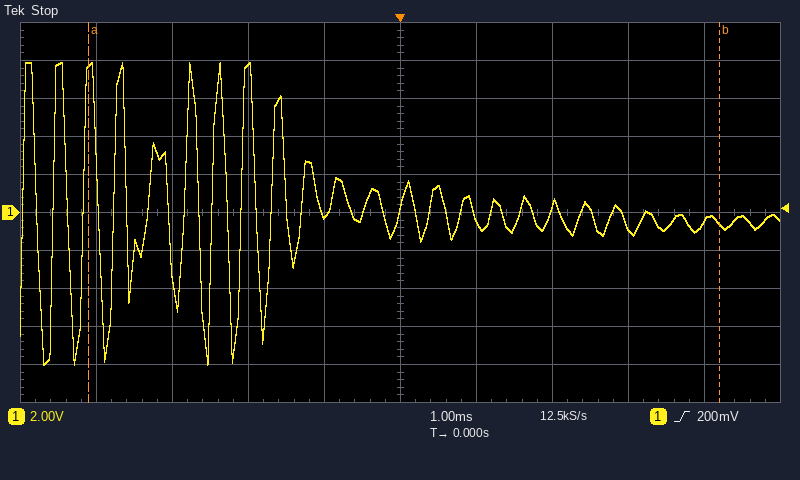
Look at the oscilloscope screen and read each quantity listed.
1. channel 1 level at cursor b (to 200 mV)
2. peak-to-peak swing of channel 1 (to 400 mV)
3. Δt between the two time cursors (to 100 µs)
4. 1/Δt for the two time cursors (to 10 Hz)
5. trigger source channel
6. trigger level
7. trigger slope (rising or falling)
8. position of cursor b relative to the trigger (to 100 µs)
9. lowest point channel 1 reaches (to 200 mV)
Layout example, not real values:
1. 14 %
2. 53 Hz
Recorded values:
1. -600 mV
2. 16.0 V
3. 8.3 ms
4. 120 Hz
5. channel 1
6. 200 mV
7. rising
8. +4.2 ms
9. -8.0 V
